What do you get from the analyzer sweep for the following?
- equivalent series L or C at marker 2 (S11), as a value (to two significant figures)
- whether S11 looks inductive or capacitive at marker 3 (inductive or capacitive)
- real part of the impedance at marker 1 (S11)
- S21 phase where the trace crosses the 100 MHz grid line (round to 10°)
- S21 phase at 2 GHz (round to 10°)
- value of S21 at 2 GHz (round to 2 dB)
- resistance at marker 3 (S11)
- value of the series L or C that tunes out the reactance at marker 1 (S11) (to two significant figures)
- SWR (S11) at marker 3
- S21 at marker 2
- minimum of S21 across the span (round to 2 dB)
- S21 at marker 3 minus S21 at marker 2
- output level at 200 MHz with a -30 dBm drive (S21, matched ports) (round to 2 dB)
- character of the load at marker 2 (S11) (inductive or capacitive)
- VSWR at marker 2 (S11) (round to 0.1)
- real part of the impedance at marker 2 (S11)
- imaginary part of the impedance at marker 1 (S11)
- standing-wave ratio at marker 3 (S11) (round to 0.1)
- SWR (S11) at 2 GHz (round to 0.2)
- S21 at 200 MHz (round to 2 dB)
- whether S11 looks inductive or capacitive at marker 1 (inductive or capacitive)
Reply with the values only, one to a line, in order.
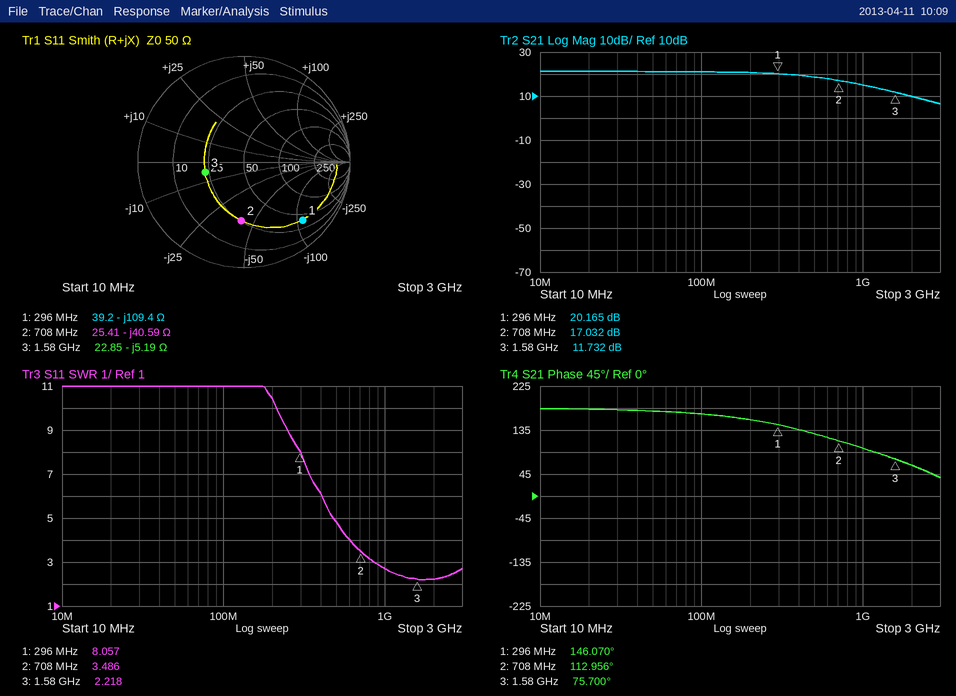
5.5 pF
capacitive
39.2 Ω
170°
60°
10 dB
22.85 Ω
59 nH
2.218
17.032 dB
6 dB
-5.300 dB
-10 dBm
capacitive
3.5
25.41 Ω
-109.4 Ω
2.2
2.2
20 dB
capacitive
